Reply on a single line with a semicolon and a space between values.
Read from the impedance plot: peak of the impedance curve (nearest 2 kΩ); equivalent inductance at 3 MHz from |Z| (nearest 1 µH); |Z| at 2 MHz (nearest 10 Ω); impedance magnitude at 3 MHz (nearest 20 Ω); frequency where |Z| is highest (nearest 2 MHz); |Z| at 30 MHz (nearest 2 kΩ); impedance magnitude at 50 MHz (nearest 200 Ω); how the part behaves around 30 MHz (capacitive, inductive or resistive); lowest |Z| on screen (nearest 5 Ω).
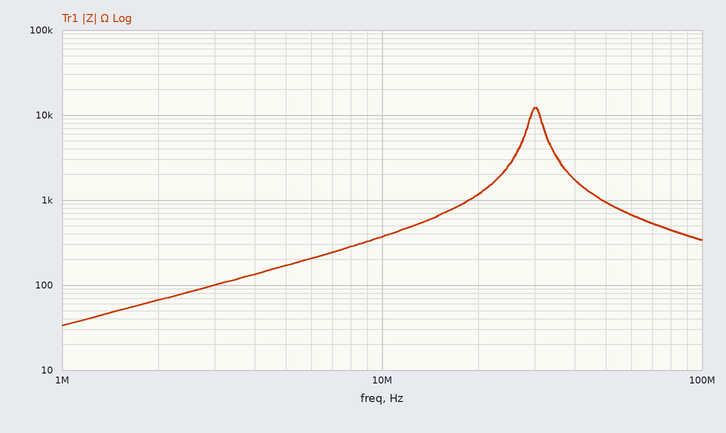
12 kΩ; 5 µH; 70 Ω; 100 Ω; 30 MHz; 12 kΩ; 1.0 kΩ; resistive; 35 Ω
